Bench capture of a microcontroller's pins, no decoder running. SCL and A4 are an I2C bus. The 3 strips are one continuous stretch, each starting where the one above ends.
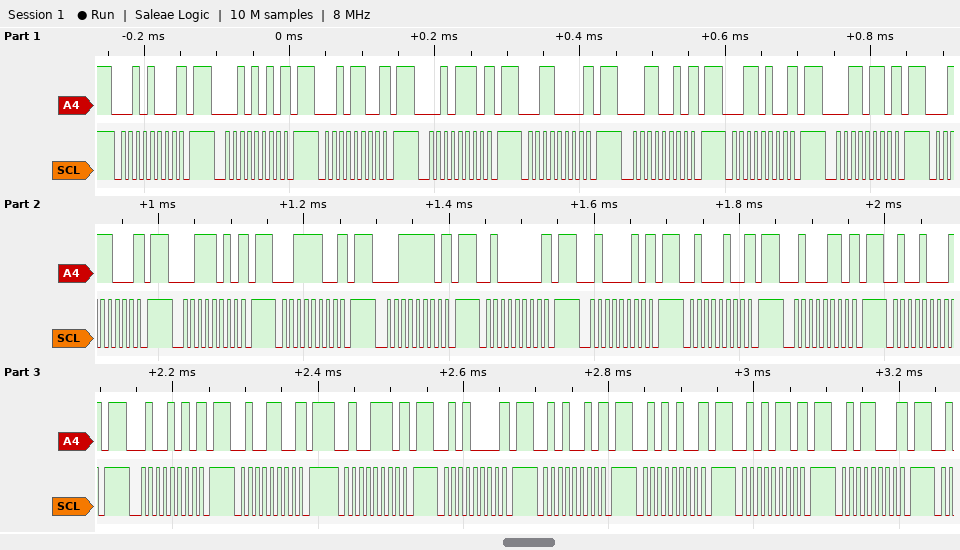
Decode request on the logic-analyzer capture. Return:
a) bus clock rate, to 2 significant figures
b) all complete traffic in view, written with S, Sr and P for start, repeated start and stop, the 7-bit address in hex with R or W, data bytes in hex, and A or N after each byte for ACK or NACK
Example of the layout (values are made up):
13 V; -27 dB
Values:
100 kHz; S 14W N P S 15W N P S 16W N P S 17W N P S 18W N P S 19W N P S 1AW N P S 1BW N P S 1CW N P S 1DW N P S 1EW N P S 1FW N P S 20W N P S 21W N P S 22W N P S 23W N P S 24W N P S 25W N P S 26W N P S 27W N P S 28W N P S 29W N P S 2AW N P S 2BW N P S 2CW N P
